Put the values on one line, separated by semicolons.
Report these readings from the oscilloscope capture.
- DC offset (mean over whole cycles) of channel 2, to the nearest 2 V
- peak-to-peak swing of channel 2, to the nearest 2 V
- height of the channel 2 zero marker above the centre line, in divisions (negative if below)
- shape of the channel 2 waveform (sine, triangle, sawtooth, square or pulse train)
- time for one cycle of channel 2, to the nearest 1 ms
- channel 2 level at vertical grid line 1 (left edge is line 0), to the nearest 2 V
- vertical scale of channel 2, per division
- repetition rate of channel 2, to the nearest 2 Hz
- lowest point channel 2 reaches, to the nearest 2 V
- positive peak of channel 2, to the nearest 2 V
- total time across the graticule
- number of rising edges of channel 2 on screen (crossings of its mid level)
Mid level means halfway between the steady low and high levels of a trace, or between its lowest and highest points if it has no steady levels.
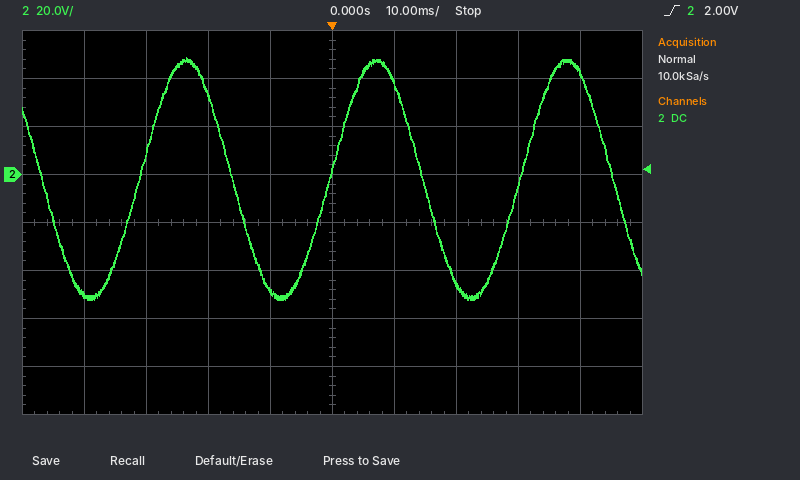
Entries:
-2 V; 100 V; +1.0 div; sine; 31 ms; -50 V; 20 V; 32 Hz; -52 V; 48 V; 100 ms; 3
